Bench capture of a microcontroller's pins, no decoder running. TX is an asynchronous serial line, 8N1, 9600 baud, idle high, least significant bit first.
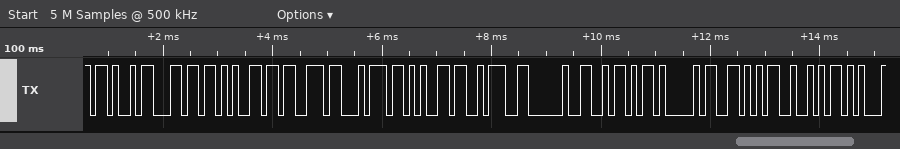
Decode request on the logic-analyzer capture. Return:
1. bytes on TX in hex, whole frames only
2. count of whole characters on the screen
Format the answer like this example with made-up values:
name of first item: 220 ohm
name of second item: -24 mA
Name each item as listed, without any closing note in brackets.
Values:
bytes on TX in hex, whole frames only: 0x4B 0x6C 0x65 0x73 0x74 0x65 0x3A 0x20 0x5A 0x41 0x56 0x52
count of whole characters on the screen: 12
